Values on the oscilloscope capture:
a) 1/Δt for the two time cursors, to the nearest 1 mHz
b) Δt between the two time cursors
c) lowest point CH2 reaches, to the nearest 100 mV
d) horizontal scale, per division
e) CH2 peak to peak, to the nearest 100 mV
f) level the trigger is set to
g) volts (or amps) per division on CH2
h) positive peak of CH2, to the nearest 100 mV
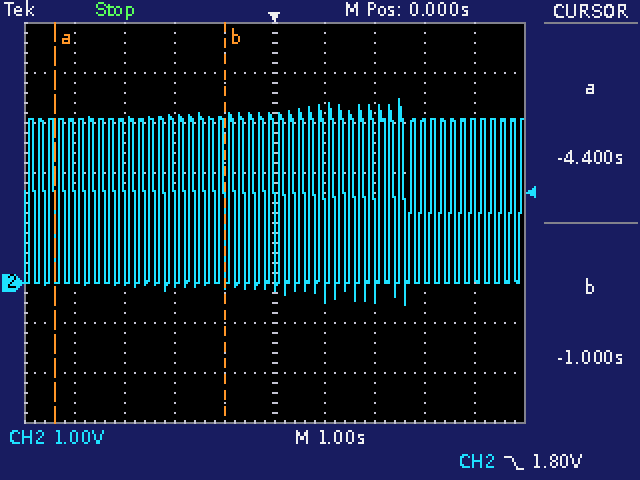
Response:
294 mHz
3.4 s
-400 mV
1 s
4.1 V
1.80 V
1 V
3.7 V
